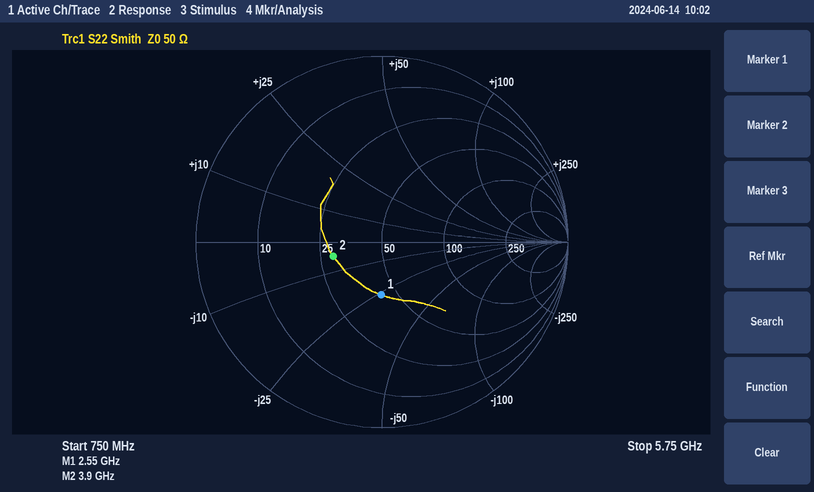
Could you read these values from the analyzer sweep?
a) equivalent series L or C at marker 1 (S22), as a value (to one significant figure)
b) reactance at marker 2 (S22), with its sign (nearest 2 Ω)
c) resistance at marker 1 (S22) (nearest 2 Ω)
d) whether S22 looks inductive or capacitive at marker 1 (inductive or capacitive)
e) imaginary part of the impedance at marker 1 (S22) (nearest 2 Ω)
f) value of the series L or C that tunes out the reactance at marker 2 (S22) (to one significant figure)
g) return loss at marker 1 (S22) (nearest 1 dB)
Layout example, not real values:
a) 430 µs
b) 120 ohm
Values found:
a) 2 pF
b) -4 Ω
c) 42 Ω
d) capacitive
e) -26 Ω
f) 200 pH
g) 11 dB
